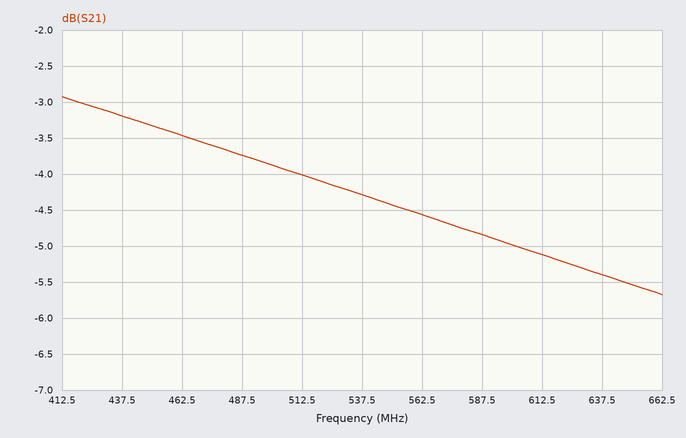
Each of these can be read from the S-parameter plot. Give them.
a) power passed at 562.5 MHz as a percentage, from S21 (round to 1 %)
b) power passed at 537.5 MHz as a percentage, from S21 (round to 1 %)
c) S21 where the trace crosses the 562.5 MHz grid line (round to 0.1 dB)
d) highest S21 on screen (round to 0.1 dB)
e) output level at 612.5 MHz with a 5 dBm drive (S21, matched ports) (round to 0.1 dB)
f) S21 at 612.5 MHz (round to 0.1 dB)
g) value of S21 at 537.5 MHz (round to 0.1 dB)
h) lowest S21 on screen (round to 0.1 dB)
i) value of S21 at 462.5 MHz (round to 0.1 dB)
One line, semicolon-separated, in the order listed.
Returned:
35 %; 37 %; -4.6 dB; -2.9 dB; -0.1 dBm; -5.1 dB; -4.3 dB; -5.7 dB; -3.5 dB
